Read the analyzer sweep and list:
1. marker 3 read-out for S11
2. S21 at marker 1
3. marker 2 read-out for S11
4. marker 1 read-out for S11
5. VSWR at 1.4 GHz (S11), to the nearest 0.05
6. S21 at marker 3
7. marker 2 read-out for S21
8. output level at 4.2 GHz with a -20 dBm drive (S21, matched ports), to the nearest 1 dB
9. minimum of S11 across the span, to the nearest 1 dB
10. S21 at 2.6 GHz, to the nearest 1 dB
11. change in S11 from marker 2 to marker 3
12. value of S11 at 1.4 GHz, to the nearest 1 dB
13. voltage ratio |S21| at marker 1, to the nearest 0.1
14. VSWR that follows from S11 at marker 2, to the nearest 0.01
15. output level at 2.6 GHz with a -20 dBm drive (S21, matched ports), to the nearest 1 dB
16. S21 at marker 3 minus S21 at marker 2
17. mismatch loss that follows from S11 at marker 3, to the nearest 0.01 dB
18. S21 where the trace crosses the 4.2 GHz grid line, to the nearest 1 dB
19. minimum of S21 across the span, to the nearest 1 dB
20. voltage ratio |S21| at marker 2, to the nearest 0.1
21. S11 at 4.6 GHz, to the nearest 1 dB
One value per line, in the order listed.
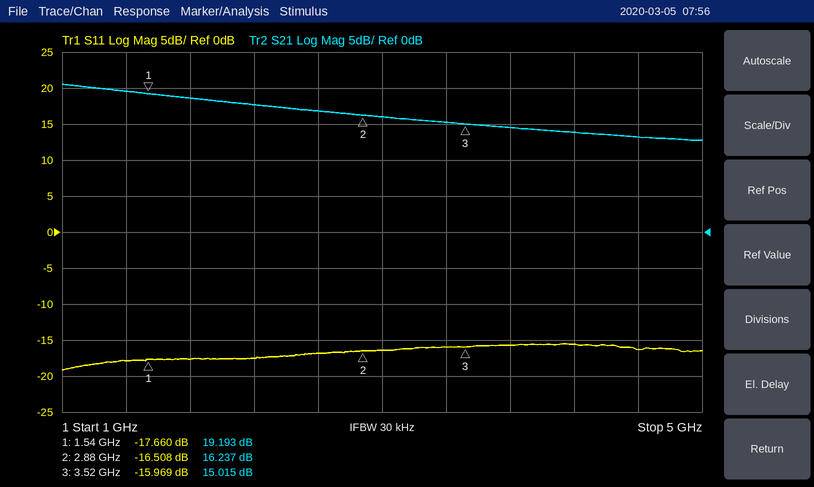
-15.969 dB
19.193 dB
-16.508 dB
-17.660 dB
1.30
15.015 dB
16.237 dB
-6 dBm
-19 dB
17 dB
0.539 dB
-18 dB
9.1
1.35
-3 dBm
-1.222 dB
0.11 dB
14 dB
13 dB
6.5
-16 dB
